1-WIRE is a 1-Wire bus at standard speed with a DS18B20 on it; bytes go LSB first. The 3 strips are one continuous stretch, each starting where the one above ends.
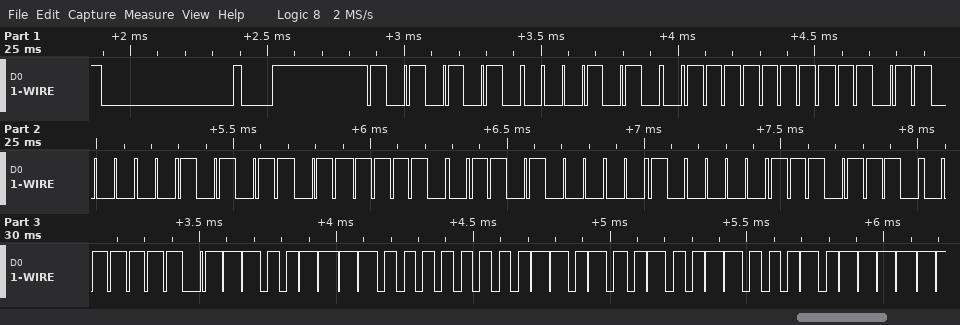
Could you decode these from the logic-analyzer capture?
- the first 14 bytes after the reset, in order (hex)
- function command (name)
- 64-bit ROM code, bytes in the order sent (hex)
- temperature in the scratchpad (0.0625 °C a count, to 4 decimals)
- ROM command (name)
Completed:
55 28 FF 1B D4 7E 16 04 77 BE F3 00 4B 46
Read Scratchpad
28 FF 1B D4 7E 16 04 77
15.1875 °C
Match ROM
